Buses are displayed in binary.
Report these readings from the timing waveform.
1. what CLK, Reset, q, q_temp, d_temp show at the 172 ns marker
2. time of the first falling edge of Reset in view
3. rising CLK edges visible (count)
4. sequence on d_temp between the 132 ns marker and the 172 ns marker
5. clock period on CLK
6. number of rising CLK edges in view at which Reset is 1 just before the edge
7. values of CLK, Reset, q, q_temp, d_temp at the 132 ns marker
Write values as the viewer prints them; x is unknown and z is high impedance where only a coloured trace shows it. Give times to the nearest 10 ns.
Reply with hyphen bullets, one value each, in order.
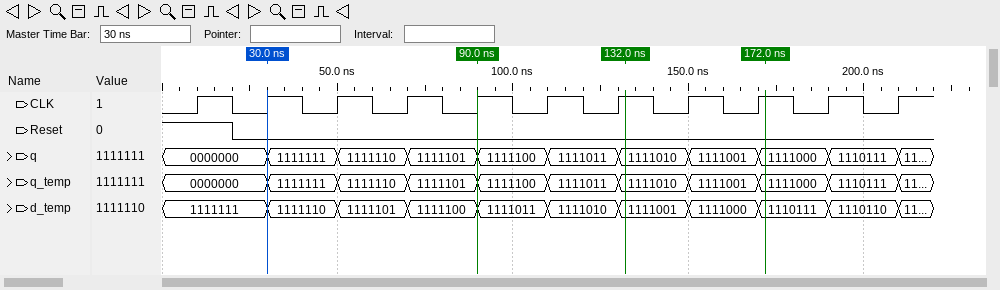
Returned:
- CLK=1, Reset=0, q=1111000, q_temp=1111000, d_temp=1110111
- 20 ns
- 11
- 1111001, 1111000, 1110111
- 20 ns
- 1
- CLK=1, Reset=0, q=1111010, q_temp=1111010, d_temp=1111001
